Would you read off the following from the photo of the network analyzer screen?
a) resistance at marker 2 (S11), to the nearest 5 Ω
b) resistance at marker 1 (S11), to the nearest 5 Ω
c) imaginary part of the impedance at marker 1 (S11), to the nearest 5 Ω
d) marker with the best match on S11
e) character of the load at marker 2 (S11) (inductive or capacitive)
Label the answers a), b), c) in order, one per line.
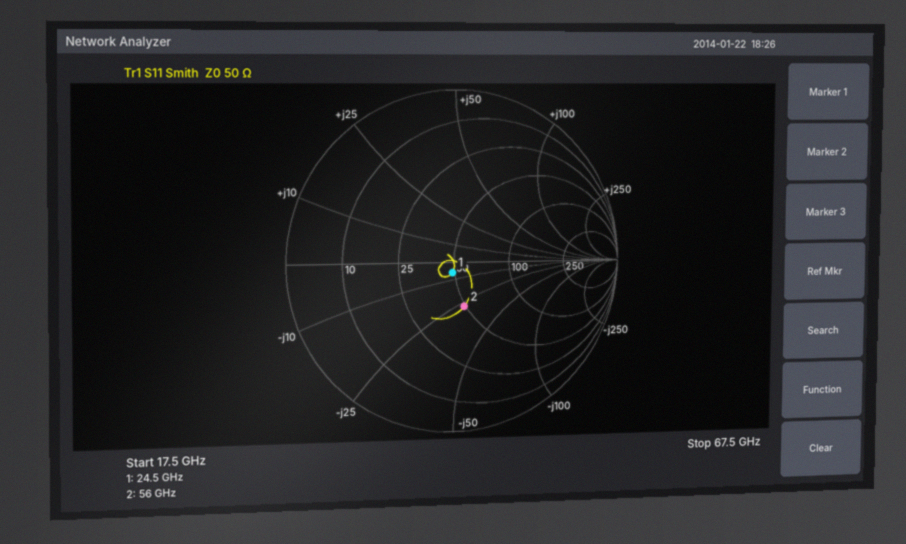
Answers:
a) 50 Ω
b) 50 Ω
c) -5 Ω
d) marker 1
e) capacitive
